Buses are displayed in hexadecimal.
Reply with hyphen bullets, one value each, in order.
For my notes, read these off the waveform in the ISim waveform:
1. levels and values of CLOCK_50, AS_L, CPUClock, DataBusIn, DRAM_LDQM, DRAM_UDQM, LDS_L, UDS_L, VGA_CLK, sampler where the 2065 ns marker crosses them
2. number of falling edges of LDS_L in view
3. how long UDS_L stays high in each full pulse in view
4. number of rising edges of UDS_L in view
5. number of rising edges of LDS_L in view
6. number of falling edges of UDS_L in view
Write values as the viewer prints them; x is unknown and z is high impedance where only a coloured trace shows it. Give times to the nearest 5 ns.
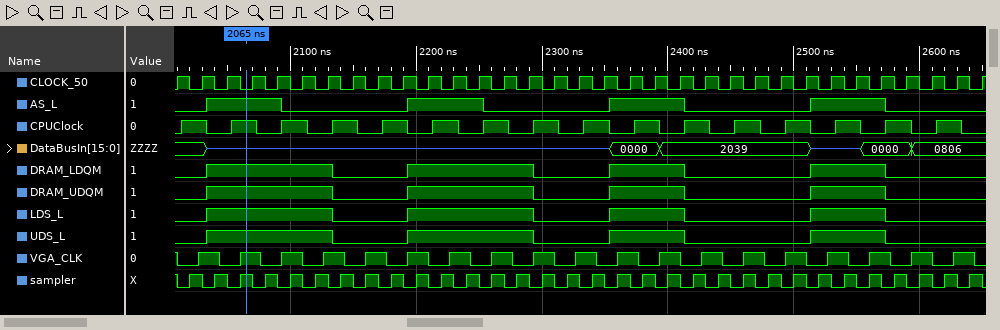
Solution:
- CLOCK_50=0, AS_L=1, CPUClock=1, DataBusIn=z, DRAM_LDQM=1, DRAM_UDQM=1, LDS_L=1, UDS_L=1, VGA_CLK=1, sampler=1
- 4
- 100 ns, 100 ns, 60 ns, 60 ns
- 4
- 4
- 4
